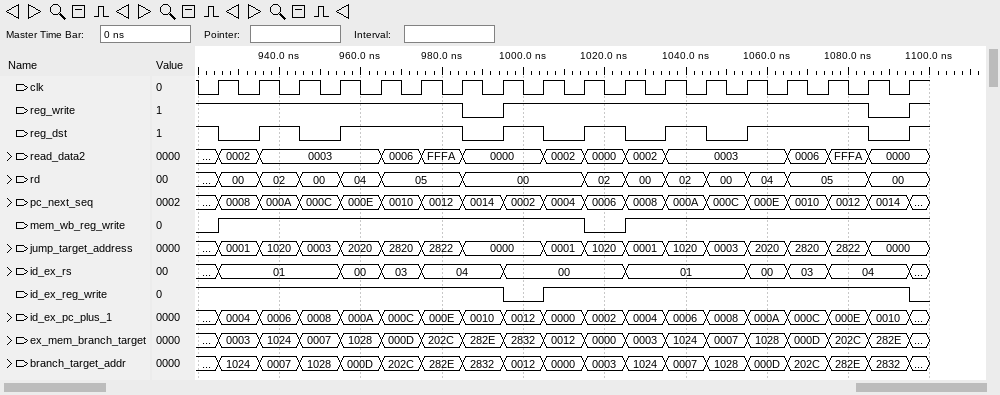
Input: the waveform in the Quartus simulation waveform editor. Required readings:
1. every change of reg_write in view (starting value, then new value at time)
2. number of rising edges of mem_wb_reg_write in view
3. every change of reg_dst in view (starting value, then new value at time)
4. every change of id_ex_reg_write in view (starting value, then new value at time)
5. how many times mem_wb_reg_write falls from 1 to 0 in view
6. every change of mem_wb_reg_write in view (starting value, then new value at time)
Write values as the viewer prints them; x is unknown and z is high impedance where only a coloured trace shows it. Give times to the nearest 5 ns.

1, 0 at 985 ns, 1 at 995 ns, 0 at 1085 ns, 1 at 1095 ns
2
1, 0 at 925 ns, 1 at 935 ns, 0 at 945 ns, 1 at 955 ns, 0 at 985 ns, 1 at 995 ns, 0 at 1005 ns, 1 at 1015 ns, 0 at 1025 ns, 1 at 1035 ns, 0 at 1045 ns, 1 at 1055 ns, 0 at 1085 ns, 1 at 1095 ns
1, 0 at 995 ns, 1 at 1005 ns, 0 at 1095 ns
1
0, 1 at 925 ns, 0 at 1015 ns, 1 at 1025 ns
